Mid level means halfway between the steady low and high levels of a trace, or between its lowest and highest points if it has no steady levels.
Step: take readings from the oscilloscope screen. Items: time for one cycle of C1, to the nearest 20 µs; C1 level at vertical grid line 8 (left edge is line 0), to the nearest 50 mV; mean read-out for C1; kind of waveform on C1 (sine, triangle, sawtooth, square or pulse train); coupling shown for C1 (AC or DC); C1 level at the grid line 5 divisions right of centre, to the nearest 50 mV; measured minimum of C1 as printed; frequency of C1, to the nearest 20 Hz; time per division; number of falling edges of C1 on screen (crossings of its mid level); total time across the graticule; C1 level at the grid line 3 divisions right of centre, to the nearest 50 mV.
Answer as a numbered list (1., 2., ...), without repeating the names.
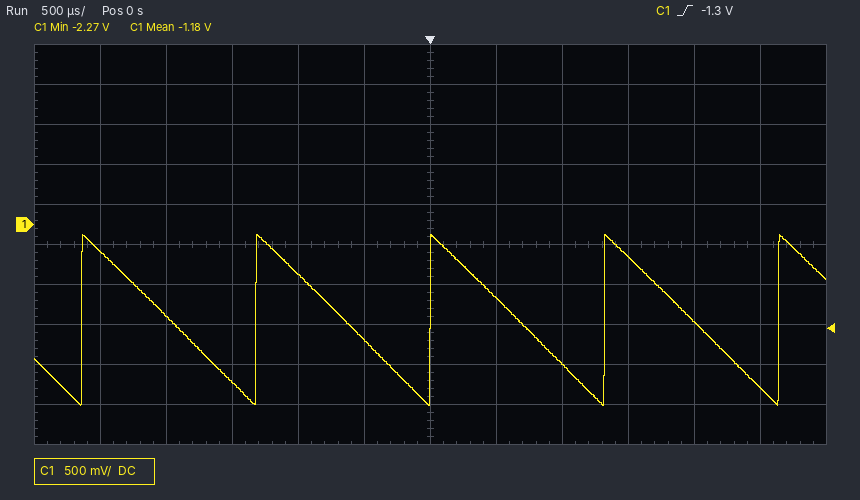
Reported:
1. 1.32 ms
2. -1.75 V
3. -1.18 V
4. sawtooth
5. DC
6. -2.05 V
7. -2.27 V
8. 760 Hz
9. 500 µs
10. 4
11. 6 ms
12. -400 mV
